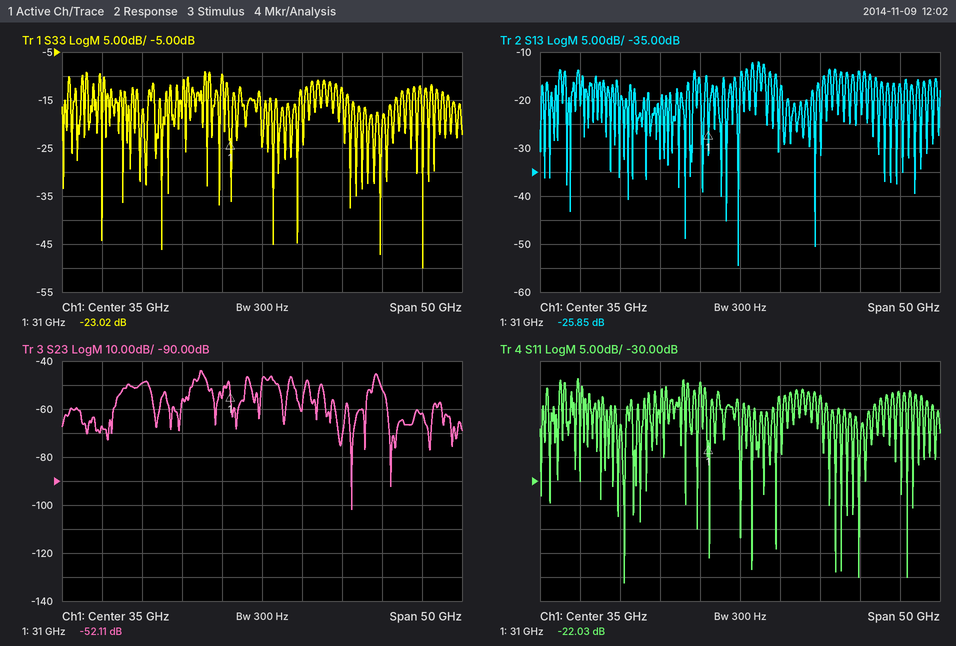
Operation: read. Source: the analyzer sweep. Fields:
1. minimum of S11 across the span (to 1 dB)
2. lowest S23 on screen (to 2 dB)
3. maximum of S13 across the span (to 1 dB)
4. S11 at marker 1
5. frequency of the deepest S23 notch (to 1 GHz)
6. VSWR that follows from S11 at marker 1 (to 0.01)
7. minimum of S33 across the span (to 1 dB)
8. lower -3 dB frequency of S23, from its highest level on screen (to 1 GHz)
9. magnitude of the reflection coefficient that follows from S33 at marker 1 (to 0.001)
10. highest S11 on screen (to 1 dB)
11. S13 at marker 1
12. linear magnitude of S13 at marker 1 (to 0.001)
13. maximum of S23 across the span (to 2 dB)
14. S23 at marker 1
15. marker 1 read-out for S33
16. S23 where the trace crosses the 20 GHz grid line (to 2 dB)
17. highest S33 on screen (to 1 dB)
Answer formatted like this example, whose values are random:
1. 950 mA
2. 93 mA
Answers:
1. -51 dB
2. -102 dB
3. -12 dB
4. -22.03 dB
5. 46 GHz
6. 1.17
7. -50 dB
8. 27 GHz
9. 0.071
10. -9 dB
11. -25.85 dB
12. 0.051
13. -44 dB
14. -52.11 dB
15. -23.02 dB
16. -50 dB
17. -9 dB
